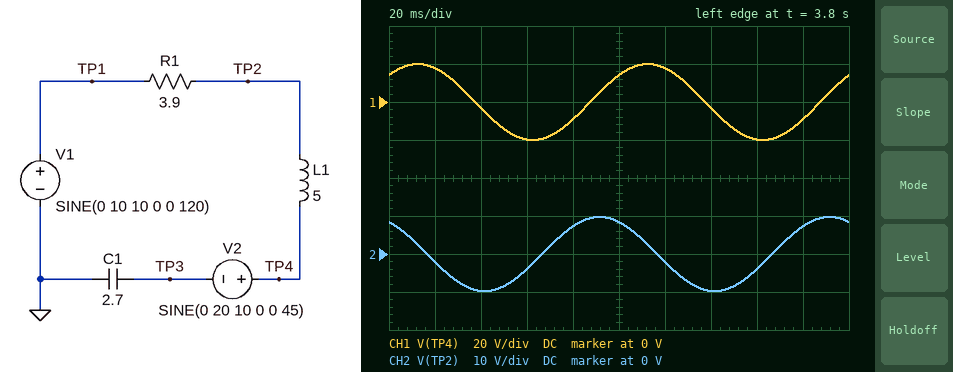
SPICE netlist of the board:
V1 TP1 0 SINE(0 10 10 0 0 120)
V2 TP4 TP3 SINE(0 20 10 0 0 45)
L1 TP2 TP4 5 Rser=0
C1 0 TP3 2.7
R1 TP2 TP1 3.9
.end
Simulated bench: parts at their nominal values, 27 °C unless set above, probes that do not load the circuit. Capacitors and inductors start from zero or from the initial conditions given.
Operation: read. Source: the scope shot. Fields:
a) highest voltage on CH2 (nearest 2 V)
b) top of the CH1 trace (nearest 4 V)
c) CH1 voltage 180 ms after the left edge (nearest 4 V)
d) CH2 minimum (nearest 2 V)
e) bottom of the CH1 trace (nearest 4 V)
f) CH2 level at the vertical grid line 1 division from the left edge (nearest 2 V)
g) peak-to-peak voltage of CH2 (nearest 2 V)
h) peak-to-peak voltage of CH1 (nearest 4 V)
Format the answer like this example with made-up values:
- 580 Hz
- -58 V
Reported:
- 10 V
- 20 V
- -8 V
- -10 V
- -20 V
- -2 V
- 20 V
- 40 V
